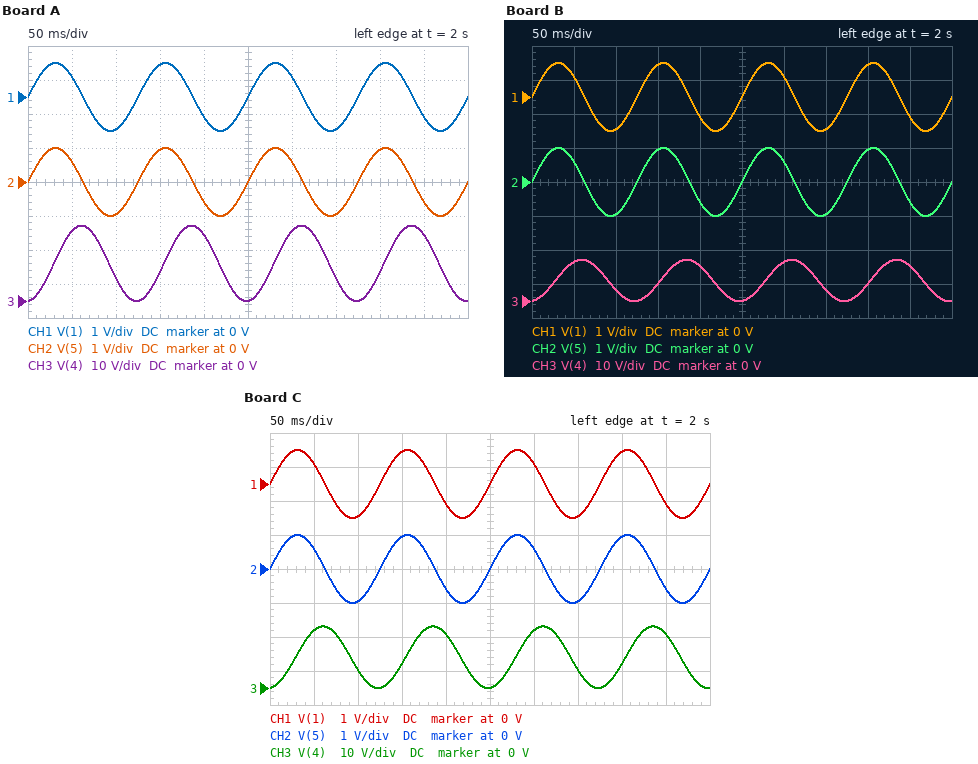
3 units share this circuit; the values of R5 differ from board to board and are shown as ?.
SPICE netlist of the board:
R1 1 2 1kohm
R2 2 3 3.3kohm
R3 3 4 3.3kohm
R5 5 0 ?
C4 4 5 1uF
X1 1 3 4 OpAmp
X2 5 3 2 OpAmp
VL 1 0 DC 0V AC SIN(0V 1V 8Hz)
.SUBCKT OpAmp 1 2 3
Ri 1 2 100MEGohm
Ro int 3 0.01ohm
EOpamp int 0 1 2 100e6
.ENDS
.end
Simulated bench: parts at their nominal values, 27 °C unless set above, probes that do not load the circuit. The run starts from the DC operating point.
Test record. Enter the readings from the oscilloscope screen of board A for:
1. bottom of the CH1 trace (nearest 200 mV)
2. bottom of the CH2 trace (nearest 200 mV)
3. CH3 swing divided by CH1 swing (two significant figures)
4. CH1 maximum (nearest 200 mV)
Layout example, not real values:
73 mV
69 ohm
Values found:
-1.0 V
-1.0 V
11
1.0 V
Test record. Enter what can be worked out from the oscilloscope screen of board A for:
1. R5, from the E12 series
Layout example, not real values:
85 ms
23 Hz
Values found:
1.8 kΩ
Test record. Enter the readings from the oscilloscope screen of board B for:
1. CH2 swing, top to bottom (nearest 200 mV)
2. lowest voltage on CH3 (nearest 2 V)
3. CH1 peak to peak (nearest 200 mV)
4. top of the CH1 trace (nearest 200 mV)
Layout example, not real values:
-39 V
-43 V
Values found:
2.0 V
0 V
2.0 V
1.0 V
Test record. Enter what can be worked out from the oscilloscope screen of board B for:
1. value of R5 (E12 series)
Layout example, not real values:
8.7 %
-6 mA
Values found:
3.3 kΩ
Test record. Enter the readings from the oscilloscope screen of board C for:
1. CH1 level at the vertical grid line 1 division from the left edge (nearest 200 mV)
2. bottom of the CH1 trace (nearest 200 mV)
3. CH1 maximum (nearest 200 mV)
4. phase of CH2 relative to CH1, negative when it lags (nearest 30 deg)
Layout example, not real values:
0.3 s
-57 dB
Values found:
600 mV
-1.0 V
1.0 V
0 deg
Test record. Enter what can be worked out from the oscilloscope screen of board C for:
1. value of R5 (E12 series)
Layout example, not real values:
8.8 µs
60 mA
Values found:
2.2 kΩ
